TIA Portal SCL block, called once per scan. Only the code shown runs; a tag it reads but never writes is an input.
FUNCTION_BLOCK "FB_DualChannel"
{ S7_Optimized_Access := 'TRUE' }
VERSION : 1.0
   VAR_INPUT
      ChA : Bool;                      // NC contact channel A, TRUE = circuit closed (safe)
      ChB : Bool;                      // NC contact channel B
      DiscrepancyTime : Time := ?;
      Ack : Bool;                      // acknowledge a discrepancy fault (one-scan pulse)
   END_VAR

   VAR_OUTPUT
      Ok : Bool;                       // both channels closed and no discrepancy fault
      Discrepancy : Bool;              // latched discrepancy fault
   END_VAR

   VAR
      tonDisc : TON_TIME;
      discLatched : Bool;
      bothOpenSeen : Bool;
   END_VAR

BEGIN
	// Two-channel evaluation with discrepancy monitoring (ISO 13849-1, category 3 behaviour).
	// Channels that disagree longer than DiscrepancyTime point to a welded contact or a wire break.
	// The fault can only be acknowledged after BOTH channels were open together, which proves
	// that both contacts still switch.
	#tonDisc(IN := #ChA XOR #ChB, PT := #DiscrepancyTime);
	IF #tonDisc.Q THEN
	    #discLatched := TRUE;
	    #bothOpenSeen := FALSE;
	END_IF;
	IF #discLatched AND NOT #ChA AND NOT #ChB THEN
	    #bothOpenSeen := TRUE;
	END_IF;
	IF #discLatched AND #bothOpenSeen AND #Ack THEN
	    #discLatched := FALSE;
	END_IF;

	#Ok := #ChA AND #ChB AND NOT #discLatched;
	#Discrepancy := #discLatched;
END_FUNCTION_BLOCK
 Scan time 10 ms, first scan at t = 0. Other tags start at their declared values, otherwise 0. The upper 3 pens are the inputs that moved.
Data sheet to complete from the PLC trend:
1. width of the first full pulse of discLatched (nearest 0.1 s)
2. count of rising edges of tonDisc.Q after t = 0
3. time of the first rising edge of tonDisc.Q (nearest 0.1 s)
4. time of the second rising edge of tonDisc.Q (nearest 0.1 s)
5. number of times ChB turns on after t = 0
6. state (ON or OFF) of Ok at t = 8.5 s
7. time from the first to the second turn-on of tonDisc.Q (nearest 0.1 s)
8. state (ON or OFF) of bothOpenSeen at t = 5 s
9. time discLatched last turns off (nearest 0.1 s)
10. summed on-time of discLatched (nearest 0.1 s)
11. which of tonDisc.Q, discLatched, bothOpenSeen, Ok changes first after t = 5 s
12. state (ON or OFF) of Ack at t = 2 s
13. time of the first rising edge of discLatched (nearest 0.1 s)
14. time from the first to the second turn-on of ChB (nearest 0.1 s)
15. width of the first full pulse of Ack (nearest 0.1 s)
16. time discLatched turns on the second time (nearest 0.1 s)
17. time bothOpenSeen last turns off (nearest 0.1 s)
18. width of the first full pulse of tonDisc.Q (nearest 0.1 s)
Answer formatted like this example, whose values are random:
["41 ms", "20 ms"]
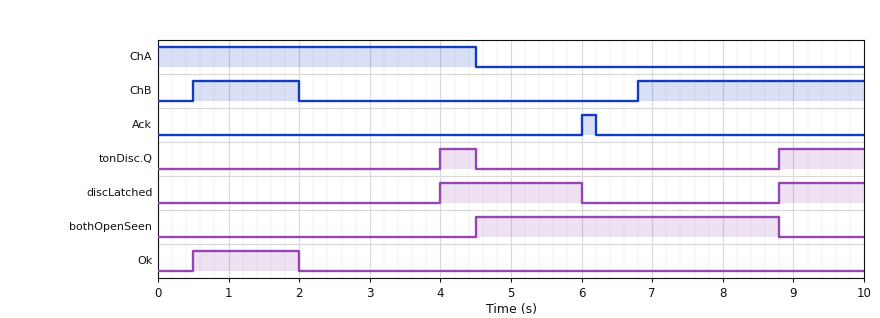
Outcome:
["2.0 s", "2", "4.0 s", "8.8 s", "2", "OFF", "4.8 s", "ON", "6.0 s", "3.2 s", "discLatched", "OFF", "4.0 s", "6.3 s", "0.2 s", "8.8 s", "8.8 s", "0.5 s"]
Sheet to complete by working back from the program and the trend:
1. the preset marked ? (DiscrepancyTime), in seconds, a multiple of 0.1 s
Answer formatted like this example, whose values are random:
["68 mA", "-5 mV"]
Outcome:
["2.0 s"]
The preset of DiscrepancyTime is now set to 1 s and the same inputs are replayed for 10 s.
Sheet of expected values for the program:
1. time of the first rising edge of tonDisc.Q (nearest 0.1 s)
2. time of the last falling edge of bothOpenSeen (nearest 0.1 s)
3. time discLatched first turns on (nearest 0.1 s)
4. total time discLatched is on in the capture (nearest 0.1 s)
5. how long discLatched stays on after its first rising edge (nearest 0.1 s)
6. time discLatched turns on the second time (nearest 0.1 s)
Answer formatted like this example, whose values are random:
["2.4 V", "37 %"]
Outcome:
["3.0 s", "7.8 s", "3.0 s", "5.2 s", "3.0 s", "7.8 s"]
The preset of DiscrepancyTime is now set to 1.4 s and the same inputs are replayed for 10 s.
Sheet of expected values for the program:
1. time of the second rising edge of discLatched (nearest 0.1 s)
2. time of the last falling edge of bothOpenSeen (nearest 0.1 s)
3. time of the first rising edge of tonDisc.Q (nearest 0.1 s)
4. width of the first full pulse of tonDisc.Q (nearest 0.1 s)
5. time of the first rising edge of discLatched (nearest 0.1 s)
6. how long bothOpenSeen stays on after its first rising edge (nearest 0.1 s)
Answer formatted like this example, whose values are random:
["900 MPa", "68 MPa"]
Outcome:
["8.2 s", "8.2 s", "3.4 s", "1.1 s", "3.4 s", "3.7 s"]
